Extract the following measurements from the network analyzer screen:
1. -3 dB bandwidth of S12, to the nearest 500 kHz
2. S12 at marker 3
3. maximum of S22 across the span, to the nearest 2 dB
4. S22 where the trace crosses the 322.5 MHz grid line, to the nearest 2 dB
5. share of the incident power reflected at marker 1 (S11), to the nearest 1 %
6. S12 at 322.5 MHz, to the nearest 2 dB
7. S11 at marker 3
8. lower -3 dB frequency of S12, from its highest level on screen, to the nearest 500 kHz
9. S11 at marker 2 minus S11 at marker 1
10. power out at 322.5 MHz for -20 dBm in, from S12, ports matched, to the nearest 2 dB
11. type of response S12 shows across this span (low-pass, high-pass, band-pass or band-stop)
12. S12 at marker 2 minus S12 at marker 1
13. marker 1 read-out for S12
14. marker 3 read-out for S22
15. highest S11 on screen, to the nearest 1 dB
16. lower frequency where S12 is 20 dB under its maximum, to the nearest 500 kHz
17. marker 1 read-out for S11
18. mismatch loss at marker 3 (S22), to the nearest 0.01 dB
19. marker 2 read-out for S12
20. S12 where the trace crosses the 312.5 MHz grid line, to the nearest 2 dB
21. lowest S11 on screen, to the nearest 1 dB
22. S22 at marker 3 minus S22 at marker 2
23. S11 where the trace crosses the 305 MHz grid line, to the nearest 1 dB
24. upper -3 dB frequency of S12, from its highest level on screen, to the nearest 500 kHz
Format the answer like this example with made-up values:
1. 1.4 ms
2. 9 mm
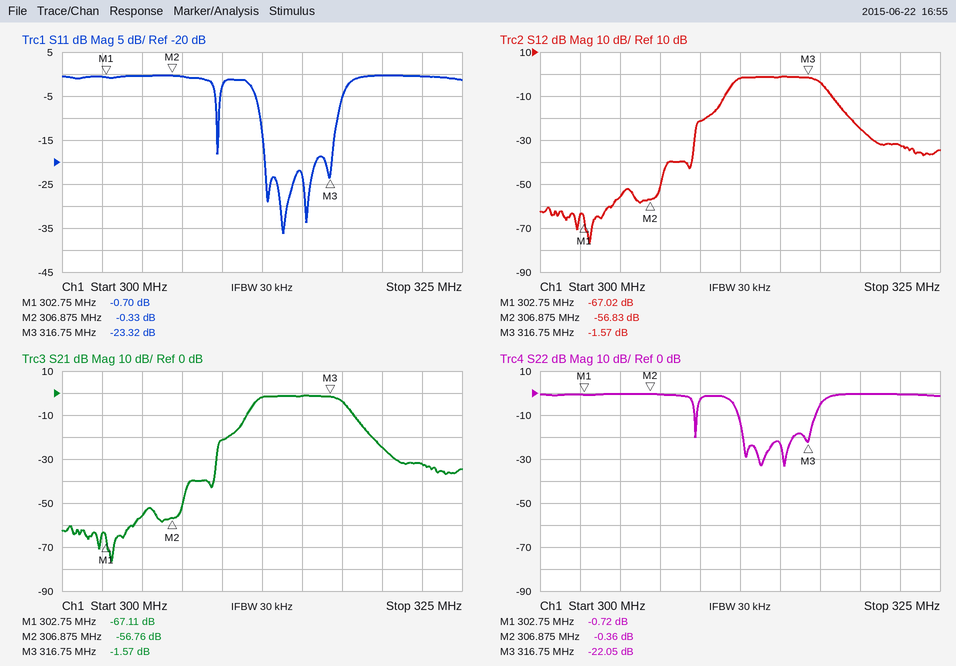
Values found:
1. 5.5 MHz
2. -1.57 dB
3. 0 dB
4. 0 dB
5. 85 %
6. -32 dB
7. -23.32 dB
8. 312.0 MHz
9. 0.37 dB
10. -52 dBm
11. band-pass
12. 10.19 dB
13. -67.02 dB
14. -22.05 dB
15. 0 dB
16. 310.0 MHz
17. -0.70 dB
18. 0.03 dB
19. -56.83 dB
20. -2 dB
21. -36 dB
22. -21.69 dB
23. 0 dB
24. 317.5 MHz
